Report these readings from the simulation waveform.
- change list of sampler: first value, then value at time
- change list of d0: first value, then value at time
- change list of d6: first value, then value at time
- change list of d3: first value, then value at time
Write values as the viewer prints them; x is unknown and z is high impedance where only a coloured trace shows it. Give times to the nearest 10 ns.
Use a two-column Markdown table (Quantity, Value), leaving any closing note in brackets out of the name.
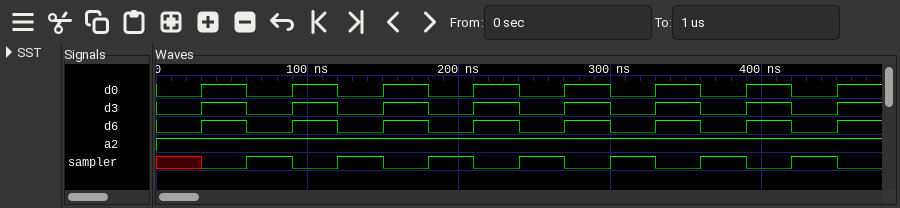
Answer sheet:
| Quantity | Value |
|---|---|
| change list of sampler: first value, then value at time | x, 0 at 30 ns, 1 at 60 ns, 0 at 90 ns, 1 at 120 ns, 0 at 150 ns, 1 at 180 ns, 0 at 210 ns, 1 at 240 ns, 0 at 270 ns, 1 at 300 ns, 0 at 330 ns, 1 at 360 ns, 0 at 390 ns, 1 at 420 ns, 0 at 450 ns |
| change list of d0: first value, then value at time | 0, 1 at 30 ns, 0 at 60 ns, 1 at 90 ns, 0 at 120 ns, 1 at 150 ns, 0 at 180 ns, 1 at 210 ns, 0 at 240 ns, 1 at 270 ns, 0 at 300 ns, 1 at 330 ns, 0 at 360 ns, 1 at 390 ns, 0 at 420 ns, 1 at 450 ns |
| change list of d6: first value, then value at time | 0, 1 at 30 ns, 0 at 60 ns, 1 at 90 ns, 0 at 120 ns, 1 at 150 ns, 0 at 180 ns, 1 at 210 ns, 0 at 240 ns, 1 at 270 ns, 0 at 300 ns, 1 at 330 ns, 0 at 360 ns, 1 at 390 ns, 0 at 420 ns, 1 at 450 ns |
| change list of d3: first value, then value at time | 0, 1 at 30 ns, 0 at 60 ns, 1 at 90 ns, 0 at 120 ns, 1 at 150 ns, 0 at 180 ns, 1 at 210 ns, 0 at 240 ns, 1 at 270 ns, 0 at 300 ns, 1 at 330 ns, 0 at 360 ns, 1 at 390 ns, 0 at 420 ns, 1 at 450 ns |
